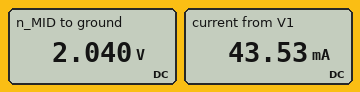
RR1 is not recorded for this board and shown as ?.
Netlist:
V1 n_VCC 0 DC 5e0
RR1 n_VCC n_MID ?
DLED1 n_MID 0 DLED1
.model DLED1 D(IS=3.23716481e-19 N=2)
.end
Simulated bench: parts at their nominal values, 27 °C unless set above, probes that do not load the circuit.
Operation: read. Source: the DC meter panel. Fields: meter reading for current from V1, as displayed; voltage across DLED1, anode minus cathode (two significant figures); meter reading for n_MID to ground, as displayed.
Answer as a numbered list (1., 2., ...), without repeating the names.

1. 43.53 mA
2. 2.0 V
3. 2.040 V
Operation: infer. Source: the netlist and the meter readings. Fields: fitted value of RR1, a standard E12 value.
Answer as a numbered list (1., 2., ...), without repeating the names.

1. 68 Ω
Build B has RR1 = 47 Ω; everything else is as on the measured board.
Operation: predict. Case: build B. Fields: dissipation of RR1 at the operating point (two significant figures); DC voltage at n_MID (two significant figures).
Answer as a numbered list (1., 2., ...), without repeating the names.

1. 180 mW
2. 2.1 V
